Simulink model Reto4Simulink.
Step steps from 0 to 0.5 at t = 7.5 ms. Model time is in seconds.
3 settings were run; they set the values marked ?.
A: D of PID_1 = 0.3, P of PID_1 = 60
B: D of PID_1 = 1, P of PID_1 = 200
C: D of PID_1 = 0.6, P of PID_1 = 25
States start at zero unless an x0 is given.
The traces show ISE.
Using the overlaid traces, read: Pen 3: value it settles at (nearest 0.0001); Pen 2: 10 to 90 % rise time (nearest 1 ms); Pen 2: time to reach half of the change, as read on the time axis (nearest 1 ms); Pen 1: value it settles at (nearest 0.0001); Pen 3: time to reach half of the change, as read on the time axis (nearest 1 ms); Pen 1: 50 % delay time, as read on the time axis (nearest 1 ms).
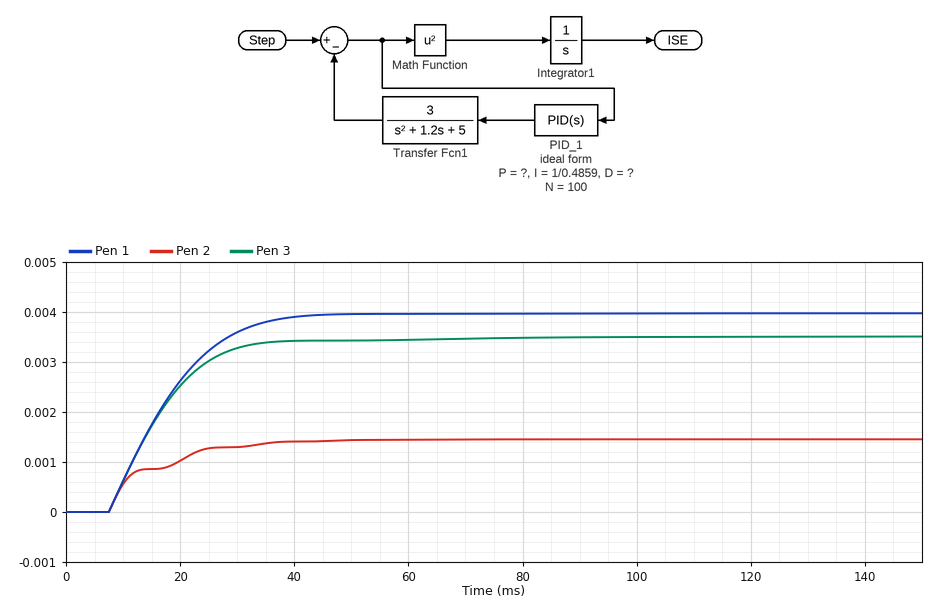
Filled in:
0.0035
23 ms
11 ms
0.0040
15 ms
16 ms
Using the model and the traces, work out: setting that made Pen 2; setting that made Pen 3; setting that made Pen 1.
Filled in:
B
A
C
